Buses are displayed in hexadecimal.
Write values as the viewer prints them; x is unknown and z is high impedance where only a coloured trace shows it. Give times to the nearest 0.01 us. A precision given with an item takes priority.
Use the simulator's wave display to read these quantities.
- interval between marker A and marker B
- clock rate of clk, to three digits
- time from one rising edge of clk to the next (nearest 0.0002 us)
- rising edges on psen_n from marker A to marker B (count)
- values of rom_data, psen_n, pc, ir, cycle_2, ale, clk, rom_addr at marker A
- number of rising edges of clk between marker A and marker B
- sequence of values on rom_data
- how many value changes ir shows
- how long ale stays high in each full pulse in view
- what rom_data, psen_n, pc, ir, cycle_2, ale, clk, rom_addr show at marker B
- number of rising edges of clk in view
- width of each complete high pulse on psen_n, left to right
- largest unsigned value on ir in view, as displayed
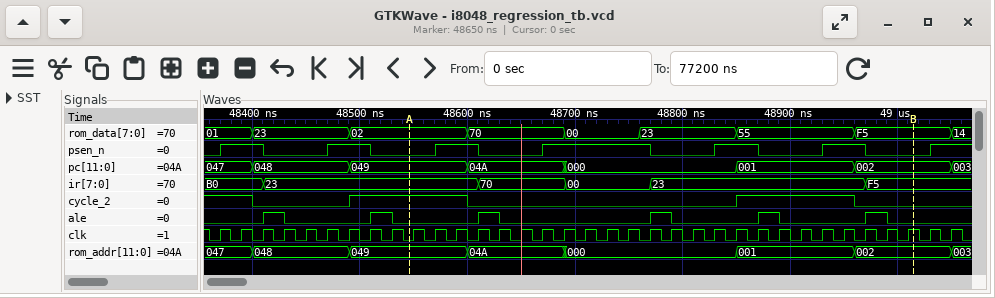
0.47 us
50.0 MHz
0.02 us
4
rom_data=02, psen_n=0, pc=049, ir=23, cycle_2=1, ale=0, clk=0, rom_addr=049
24
01, 23, 02, 70, 00, 23, 55, F5, 14
5
0.02 us, 0.02 us, 0.02 us, 0.02 us, 0.02 us, 0.02 us
rom_data=F5, psen_n=0, pc=002, ir=F5, cycle_2=0, ale=0, clk=1, rom_addr=002
35
0.04 us, 0.04 us, 0.04 us, 0.1 us, 0.04 us, 0.04 us
F5
